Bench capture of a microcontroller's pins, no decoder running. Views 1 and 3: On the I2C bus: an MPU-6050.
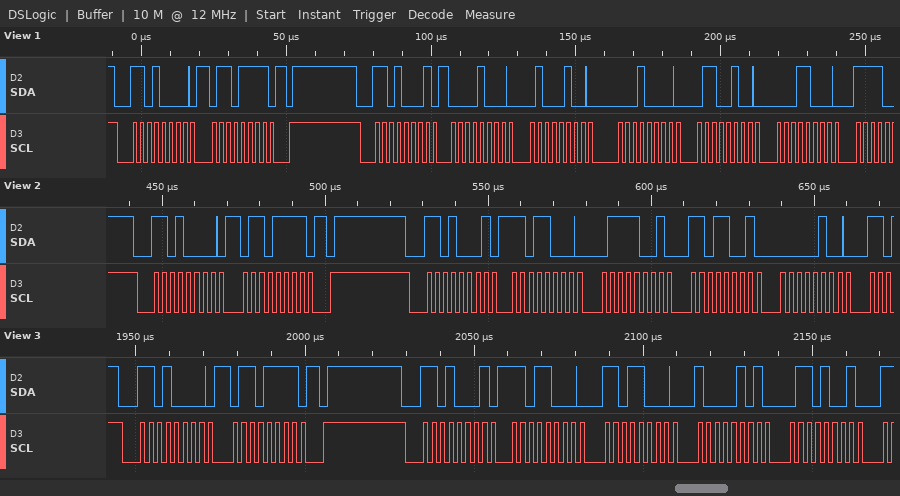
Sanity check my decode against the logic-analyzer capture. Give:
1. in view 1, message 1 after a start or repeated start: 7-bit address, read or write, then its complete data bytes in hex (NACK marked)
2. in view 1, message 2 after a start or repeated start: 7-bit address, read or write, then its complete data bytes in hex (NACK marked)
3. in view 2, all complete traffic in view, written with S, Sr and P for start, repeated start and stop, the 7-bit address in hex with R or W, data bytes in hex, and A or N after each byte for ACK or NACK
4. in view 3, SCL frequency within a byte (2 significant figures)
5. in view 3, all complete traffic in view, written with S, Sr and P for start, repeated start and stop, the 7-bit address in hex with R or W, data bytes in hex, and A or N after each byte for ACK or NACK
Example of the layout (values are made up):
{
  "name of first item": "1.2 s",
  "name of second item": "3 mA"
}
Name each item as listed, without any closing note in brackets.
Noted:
{
  "in view 1, message 1 after a start or repeated start: 7-bit address, read or write, then its complete data bytes in hex": "0x68 write: 6F",
  "in view 1, message 2 after a start or repeated start: 7-bit address, read or write, then its complete data bytes in hex": "0x68 read: 08 44 10 64 18",
  "in view 2, all complete traffic in view, written with S, Sr and P for start, repeated start and stop, the 7-bit address in hex with R or W, data bytes in hex, and A or N after each byte for ACK or NACK": "S 68W A 6F A P S 68R A D8 A 79 A D9 A 04 A",
  "in view 3, SCL frequency within a byte": "400 kHz",
  "in view 3, all complete traffic in view, written with S, Sr and P for start, repeated start and stop, the 7-bit address in hex with R or W, data bytes in hex, and A or N after each byte for ACK or NACK": "S 68W A 6F A P S 68R A D8 A D8 A 85 A 69 A"
}
